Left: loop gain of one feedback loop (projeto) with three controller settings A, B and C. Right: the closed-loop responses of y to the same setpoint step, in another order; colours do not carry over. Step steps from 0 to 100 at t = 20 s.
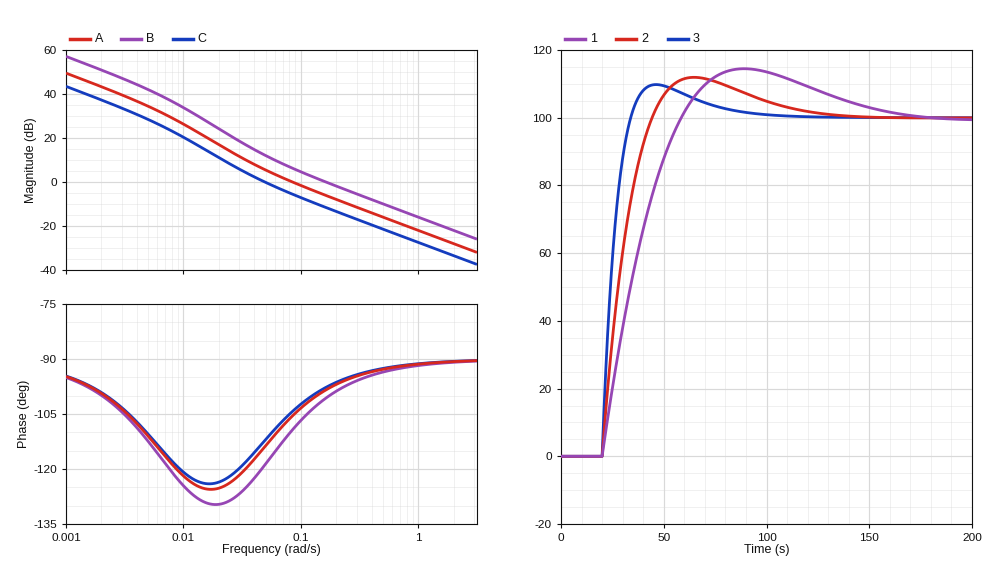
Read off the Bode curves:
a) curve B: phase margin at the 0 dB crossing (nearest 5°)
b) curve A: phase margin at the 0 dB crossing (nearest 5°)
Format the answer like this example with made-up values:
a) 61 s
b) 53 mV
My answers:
a) 80°
b) 75°
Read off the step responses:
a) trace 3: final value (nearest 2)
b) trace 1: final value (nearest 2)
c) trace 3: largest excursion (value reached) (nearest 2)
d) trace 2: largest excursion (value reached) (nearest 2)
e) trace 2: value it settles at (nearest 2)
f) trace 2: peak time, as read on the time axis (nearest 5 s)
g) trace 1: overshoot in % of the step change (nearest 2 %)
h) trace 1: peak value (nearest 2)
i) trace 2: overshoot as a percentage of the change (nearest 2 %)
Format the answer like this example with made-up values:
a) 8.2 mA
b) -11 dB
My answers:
a) 100
b) 100
c) 110
d) 112
e) 100
f) 65 s
g) 14 %
h) 114
i) 12 %
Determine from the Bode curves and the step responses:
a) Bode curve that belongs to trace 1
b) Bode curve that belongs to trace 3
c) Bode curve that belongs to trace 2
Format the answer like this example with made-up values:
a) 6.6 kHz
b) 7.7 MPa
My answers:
a) C
b) B
c) A
